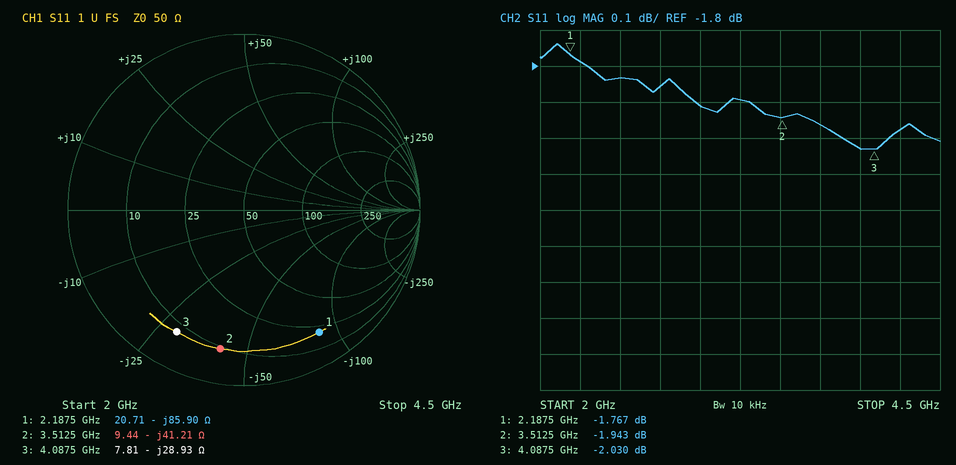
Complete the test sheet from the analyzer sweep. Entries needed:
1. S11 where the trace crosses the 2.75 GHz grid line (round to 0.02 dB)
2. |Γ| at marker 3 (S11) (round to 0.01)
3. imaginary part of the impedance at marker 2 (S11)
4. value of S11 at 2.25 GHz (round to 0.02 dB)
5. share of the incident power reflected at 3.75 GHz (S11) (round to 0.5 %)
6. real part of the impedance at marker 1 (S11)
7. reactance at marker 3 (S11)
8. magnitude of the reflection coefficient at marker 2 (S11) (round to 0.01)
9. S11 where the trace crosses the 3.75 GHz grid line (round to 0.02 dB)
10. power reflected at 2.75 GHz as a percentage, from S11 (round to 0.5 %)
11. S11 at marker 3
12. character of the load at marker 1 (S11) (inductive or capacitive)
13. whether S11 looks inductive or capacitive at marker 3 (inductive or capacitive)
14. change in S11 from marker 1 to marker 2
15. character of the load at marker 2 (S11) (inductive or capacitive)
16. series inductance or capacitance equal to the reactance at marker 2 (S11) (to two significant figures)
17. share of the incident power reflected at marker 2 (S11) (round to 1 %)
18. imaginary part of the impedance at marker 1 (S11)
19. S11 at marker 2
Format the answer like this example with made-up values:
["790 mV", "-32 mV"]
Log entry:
["-1.86 dB", "0.79", "-41.21 Ω", "-1.78 dB", "63.5 %", "20.71 Ω", "-28.93 Ω", "0.80", "-1.96 dB", "65.0 %", "-2.030 dB", "capacitive", "capacitive", "-0.176 dB", "capacitive", "1.1 pF", "64 %", "-85.90 Ω", "-1.943 dB"]
